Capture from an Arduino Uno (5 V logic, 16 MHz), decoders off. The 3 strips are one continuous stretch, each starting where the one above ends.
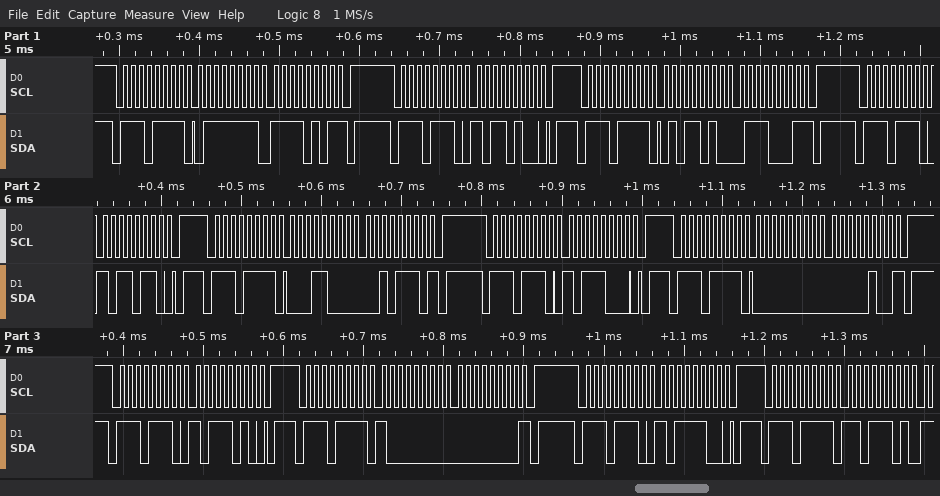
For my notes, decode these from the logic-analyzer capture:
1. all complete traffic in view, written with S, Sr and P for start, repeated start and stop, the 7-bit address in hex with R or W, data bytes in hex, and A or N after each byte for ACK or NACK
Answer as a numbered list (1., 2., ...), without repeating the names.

1. S 77R A 7F A F5 N P S 77W A B4 A P S 77R A 5A A 71 N P S 77W A B6 A P S 77R A 18 A 2E N P S 77W A B8 A P S 77R A 00 A 04 N P S 77W A BA A P S 77R A 80 A 00 N P S 77W A BC A P S 77R A DD A
